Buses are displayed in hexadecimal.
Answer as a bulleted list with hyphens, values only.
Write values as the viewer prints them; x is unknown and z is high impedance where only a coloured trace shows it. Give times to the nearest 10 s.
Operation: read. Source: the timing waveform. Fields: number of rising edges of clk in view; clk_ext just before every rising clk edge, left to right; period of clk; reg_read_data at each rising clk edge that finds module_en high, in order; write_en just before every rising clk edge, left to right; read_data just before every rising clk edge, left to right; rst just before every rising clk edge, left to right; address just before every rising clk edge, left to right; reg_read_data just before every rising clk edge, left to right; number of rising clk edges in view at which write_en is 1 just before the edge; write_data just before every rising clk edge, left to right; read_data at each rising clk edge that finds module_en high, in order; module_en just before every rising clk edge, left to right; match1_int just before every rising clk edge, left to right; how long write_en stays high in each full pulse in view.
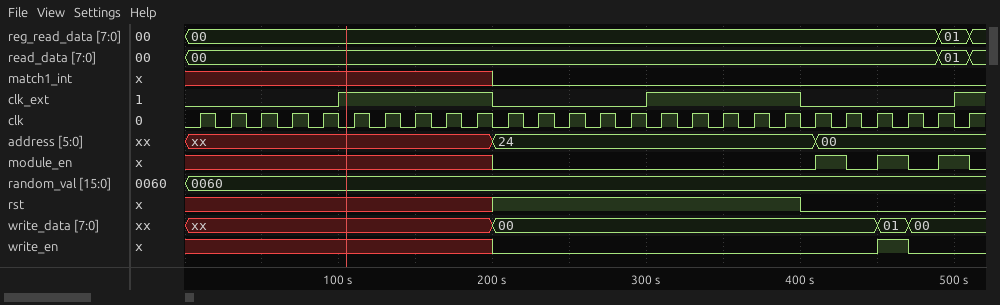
- 26
- 0 0 0 0 0 1 1 1 1 1 0 0 0 0 0 1 1 1 1 1 0 0 0 0 0 1
- 20 s
- 00, 00, 01
- x x x x x x x x x x 0 0 0 0 0 0 0 0 0 0 0 0 0 1 0 0
- 00, 00, 00, 00, 00, 00, 00, 00, 00, 00, 00, 00, 00, 00, 00, 00, 00, 00, 00, 00, 00, 00, 00, 00, 00, 01
- x x x x x x x x x x 1 1 1 1 1 1 1 1 1 1 0 0 0 0 0 0
- xx, xx, xx, xx, xx, xx, xx, xx, xx, xx, 24, 24, 24, 24, 24, 24, 24, 24, 24, 24, 24, 00, 00, 00, 00, 00
- 00, 00, 00, 00, 00, 00, 00, 00, 00, 00, 00, 00, 00, 00, 00, 00, 00, 00, 00, 00, 00, 00, 00, 00, 00, 01
- 1
- xx, xx, xx, xx, xx, xx, xx, xx, xx, xx, 00, 00, 00, 00, 00, 00, 00, 00, 00, 00, 00, 00, 00, 01, 00, 00
- 00, 00, 01
- x x x x x x x x x x 0 0 0 0 0 0 0 0 0 0 0 1 0 1 0 1
- x x x x x x x x x x 0 0 0 0 0 0 0 0 0 0 0 0 0 0 0 0
- 20 s
